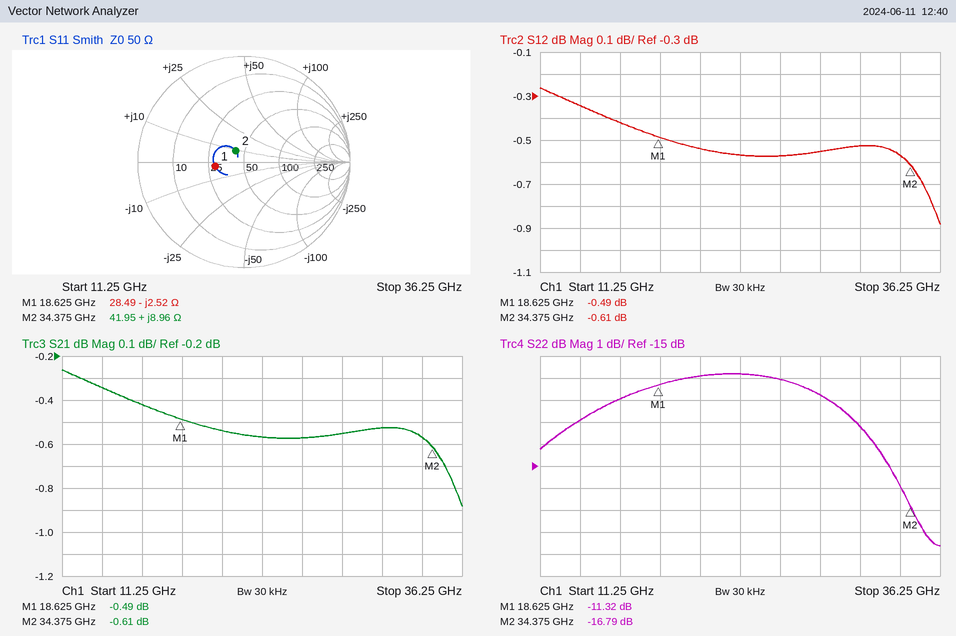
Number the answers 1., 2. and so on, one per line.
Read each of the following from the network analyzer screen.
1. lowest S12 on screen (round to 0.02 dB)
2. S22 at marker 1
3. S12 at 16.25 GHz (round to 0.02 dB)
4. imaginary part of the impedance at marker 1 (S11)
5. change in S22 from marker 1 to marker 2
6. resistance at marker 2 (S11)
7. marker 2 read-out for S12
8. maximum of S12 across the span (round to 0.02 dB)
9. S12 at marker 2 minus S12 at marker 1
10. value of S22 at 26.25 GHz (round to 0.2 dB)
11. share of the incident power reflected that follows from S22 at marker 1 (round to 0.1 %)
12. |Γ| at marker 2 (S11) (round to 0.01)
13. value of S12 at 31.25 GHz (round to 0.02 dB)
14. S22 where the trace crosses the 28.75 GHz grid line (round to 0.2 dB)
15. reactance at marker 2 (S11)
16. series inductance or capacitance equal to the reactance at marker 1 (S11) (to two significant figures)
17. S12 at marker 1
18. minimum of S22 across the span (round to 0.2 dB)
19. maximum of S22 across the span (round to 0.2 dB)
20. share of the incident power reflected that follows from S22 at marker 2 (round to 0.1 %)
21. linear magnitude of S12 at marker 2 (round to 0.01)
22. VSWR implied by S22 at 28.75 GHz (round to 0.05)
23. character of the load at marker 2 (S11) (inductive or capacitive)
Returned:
1. -0.88 dB
2. -11.32 dB
3. -0.42 dB
4. -2.52 Ω
5. -5.47 dB
6. 41.95 Ω
7. -0.61 dB
8. -0.26 dB
9. -0.12 dB
10. -11.0 dB
11. 7.4 %
12. 0.13
13. -0.52 dB
14. -11.8 dB
15. +8.96 Ω
16. 3.4 pF
17. -0.49 dB
18. -18.6 dB
19. -10.8 dB
20. 2.1 %
21. 0.93
22. 1.70
23. inductive
